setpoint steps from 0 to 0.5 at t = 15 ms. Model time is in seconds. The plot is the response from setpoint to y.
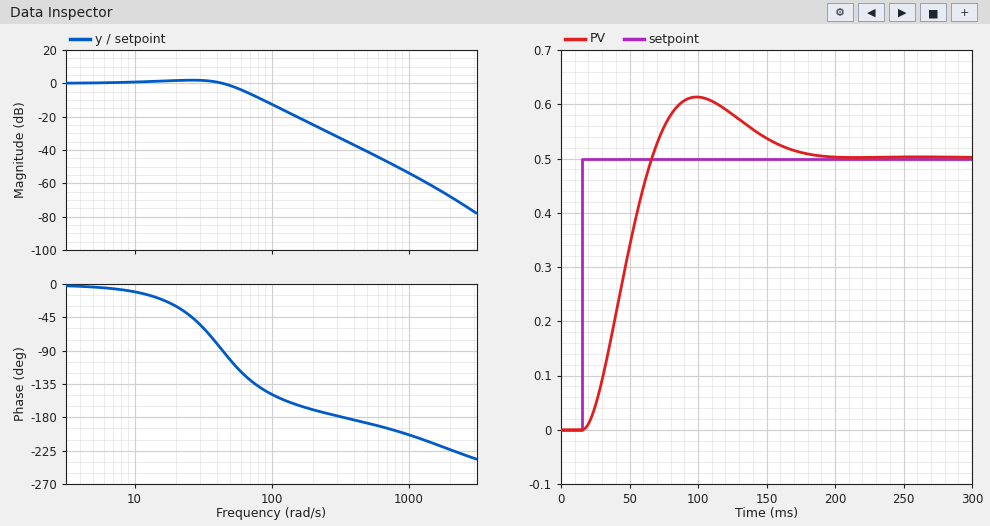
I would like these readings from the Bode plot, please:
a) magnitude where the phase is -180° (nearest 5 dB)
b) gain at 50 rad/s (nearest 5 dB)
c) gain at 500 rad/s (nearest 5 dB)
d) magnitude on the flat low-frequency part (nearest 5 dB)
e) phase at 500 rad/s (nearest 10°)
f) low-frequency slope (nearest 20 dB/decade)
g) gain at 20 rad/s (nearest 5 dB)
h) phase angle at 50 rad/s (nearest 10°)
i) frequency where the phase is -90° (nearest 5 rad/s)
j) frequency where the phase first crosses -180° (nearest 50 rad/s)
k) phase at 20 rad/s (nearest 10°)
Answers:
-35 dB
0 dB
-40 dB
0 dB
-190°
0 dB/decade
0 dB
-100°
45 rad/s
350 rad/s
-30°
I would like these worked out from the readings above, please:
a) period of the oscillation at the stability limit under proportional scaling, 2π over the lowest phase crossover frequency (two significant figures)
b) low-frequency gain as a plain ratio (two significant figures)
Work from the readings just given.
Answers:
0.018 s
1.0
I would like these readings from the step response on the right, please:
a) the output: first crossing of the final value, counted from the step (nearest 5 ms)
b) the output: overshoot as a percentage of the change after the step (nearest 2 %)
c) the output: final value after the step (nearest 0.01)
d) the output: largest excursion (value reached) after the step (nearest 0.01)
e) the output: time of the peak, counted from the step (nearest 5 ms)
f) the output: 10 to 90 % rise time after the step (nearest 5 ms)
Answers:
50 ms
22 %
0.50
0.61
85 ms
35 ms
